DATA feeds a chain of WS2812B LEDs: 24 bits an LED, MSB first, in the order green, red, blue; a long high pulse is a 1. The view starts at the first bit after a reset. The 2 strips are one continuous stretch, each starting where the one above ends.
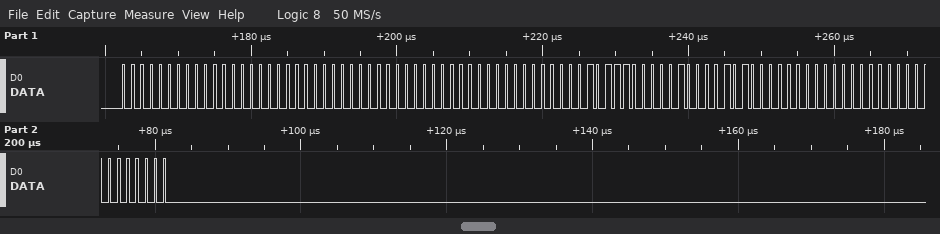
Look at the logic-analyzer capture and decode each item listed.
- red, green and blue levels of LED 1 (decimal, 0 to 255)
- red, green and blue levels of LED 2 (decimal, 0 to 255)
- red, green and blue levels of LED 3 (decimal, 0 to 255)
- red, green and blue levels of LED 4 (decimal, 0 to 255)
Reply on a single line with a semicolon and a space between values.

0, 0, 0; 0, 0, 0; 4, 23, 40; 0, 0, 0
